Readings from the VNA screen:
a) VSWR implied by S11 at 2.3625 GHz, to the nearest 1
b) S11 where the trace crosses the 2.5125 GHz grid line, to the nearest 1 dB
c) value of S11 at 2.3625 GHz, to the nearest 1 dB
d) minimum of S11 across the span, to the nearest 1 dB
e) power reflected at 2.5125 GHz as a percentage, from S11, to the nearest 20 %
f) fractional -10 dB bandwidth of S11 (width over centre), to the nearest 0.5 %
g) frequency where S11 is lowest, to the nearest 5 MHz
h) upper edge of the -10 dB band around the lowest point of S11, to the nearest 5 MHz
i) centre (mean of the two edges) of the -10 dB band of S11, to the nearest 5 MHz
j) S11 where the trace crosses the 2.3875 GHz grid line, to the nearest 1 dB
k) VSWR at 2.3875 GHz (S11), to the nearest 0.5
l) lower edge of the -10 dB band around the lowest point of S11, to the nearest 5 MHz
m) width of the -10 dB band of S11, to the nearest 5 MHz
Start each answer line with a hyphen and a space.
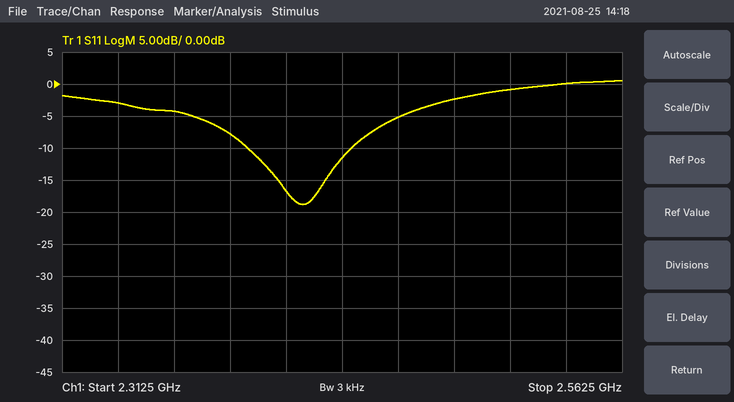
- 4
- -1 dB
- -4 dB
- -19 dB
- 80 %
- 2.0 %
- 2.420 GHz
- 2.440 GHz
- 2.420 GHz
- -8 dB
- 2.5
- 2.395 GHz
- 45 MHz
